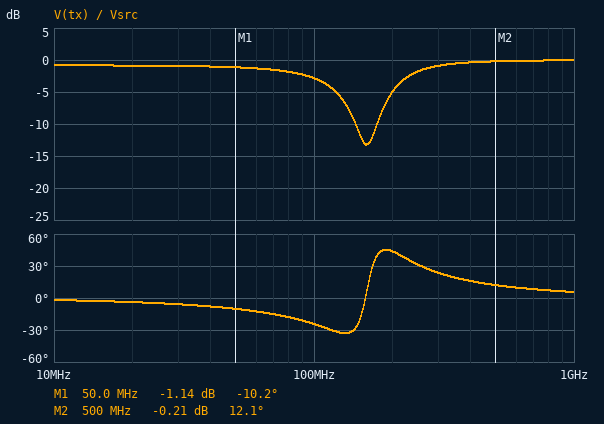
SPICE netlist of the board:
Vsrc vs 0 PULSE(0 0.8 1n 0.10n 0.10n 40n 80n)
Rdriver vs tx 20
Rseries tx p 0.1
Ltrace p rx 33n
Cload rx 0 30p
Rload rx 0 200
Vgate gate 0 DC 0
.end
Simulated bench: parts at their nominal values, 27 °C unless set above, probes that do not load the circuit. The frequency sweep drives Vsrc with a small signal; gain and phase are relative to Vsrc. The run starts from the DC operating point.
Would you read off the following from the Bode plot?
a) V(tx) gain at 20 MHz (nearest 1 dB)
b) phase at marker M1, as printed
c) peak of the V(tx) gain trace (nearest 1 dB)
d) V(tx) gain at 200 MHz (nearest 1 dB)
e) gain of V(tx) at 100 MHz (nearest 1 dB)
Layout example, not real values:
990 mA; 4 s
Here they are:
-1 dB; -10.2 deg; 0 dB; -5 dB; -3 dB
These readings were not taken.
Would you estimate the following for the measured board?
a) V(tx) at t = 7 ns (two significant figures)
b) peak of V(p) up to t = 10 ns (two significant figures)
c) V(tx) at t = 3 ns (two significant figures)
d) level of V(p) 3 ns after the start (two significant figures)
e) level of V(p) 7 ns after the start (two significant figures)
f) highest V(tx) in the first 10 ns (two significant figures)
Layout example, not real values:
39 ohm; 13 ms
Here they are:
750 mV; 800 mV; 510 mV; 510 mV; 750 mV; 800 mV
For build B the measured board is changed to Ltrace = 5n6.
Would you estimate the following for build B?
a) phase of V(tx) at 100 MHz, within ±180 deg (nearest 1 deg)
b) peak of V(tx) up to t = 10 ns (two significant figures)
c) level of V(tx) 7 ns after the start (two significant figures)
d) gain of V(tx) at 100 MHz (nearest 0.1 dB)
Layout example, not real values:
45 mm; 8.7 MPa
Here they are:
-20 deg; 740 mV; 730 mV; -1.5 dB
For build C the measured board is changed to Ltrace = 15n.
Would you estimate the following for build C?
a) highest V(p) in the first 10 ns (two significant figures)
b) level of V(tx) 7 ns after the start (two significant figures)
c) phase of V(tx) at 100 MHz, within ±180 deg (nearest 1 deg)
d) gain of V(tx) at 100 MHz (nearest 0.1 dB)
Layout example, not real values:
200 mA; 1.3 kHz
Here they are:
790 mV; 720 mV; -21 deg; -1.8 dB
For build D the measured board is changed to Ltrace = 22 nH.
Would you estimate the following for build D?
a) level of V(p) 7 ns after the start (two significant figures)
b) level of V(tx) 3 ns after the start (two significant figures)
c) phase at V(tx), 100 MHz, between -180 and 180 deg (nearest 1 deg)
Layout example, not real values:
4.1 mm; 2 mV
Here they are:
710 mV; 560 mV; -23 deg
